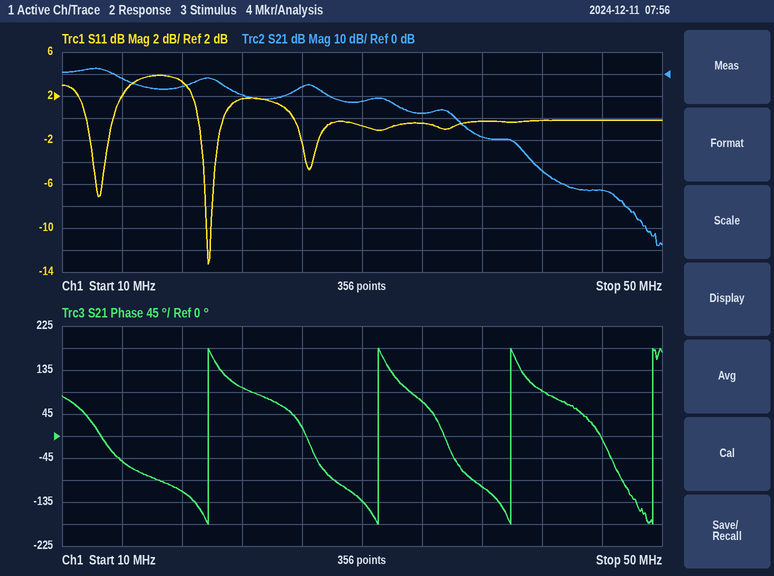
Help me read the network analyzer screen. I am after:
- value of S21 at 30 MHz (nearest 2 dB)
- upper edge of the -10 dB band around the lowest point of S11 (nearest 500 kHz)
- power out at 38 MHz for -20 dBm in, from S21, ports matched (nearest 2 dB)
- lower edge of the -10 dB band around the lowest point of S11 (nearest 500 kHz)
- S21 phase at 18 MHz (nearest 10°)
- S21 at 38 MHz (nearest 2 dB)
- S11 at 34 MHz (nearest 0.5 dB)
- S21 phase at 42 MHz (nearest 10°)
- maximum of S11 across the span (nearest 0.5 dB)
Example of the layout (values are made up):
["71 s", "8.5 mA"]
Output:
["-12 dB", "20.0 MHz", "-48 dBm", "19.5 MHz", "-110°", "-28 dB", "-0.5 dB", "90°", "4.0 dB"]
